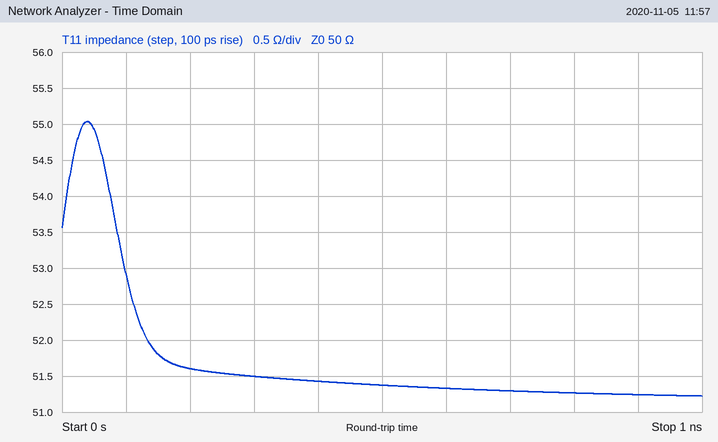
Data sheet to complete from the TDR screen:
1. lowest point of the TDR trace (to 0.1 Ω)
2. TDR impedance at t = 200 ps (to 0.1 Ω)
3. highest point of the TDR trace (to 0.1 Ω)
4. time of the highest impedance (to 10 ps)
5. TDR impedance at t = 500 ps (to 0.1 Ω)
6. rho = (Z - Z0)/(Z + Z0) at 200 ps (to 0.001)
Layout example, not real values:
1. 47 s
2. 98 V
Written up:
1. 51.2 Ω
2. 51.6 Ω
3. 55.0 Ω
4. 40 ps
5. 51.4 Ω
6. +0.016
